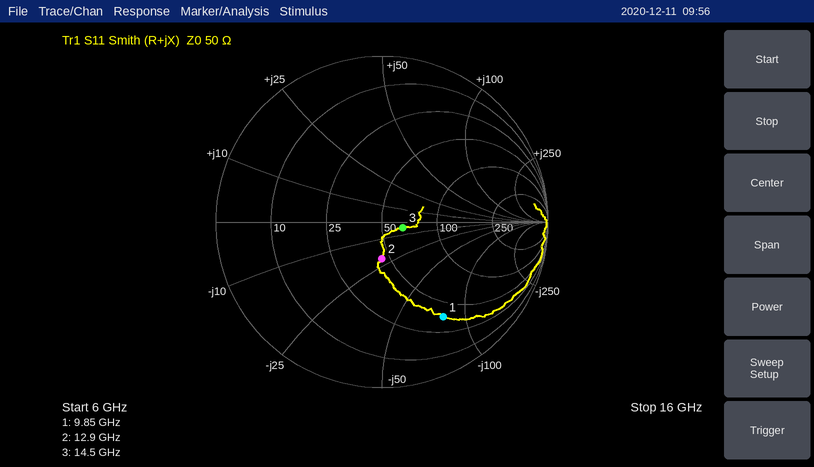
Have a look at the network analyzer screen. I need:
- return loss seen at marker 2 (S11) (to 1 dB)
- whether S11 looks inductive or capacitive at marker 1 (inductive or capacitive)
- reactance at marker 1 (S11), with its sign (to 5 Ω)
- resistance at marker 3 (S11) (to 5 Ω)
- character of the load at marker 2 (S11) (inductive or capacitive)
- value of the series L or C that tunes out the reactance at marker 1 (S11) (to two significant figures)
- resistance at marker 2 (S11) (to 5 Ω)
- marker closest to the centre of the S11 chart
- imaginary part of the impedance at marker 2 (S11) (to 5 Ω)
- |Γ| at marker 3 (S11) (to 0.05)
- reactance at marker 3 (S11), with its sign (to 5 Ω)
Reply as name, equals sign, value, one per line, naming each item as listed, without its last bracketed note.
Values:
return loss seen at marker 2 (S11) = 13 dB
whether S11 looks inductive or capacitive at marker 1 = capacitive
reactance at marker 1 (S11), with its sign = -80 Ω
resistance at marker 3 (S11) = 65 Ω
character of the load at marker 2 (S11) = capacitive
value of the series L or C that tunes out the reactance at marker 1 (S11) = 1.3 nH
resistance at marker 2 (S11) = 45 Ω
marker closest to the centre of the S11 chart = marker 3
imaginary part of the impedance at marker 2 (S11) = -20 Ω
|Γ| at marker 3 (S11) = 0.15
reactance at marker 3 (S11), with its sign = -5 Ω
